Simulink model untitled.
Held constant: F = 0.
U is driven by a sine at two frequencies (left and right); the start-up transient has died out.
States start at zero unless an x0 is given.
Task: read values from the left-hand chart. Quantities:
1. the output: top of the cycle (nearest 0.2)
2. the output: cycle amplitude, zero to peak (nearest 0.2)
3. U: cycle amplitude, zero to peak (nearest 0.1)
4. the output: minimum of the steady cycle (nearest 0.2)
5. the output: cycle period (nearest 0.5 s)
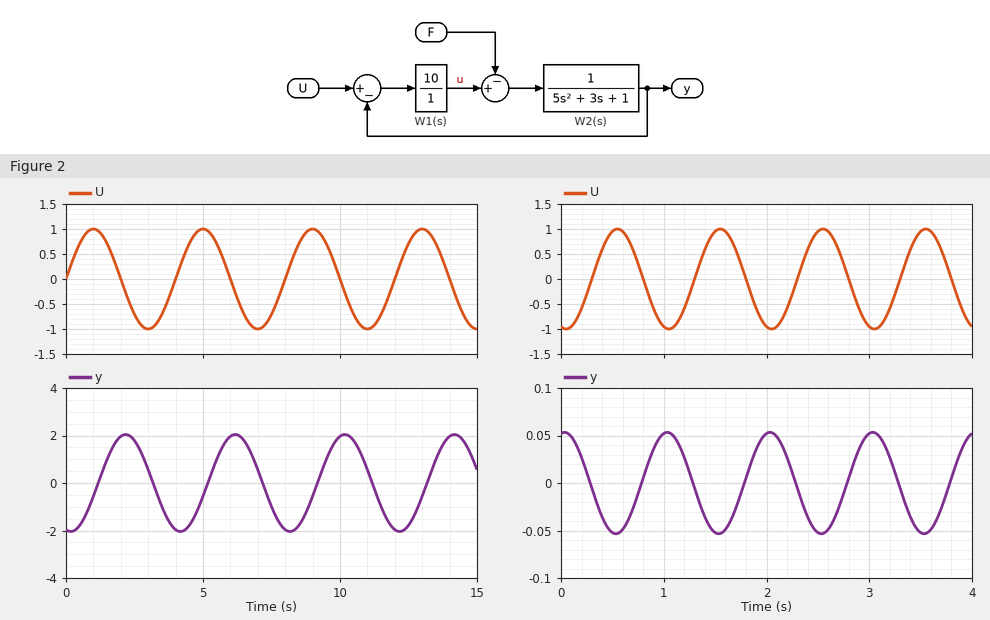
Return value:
2.0
2.0
1.0
-2.0
4.0 s
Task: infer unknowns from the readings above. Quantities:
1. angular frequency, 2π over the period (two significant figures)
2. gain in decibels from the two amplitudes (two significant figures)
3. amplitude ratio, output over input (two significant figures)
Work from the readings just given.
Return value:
1.6 rad/s
6.0 dB
2.0
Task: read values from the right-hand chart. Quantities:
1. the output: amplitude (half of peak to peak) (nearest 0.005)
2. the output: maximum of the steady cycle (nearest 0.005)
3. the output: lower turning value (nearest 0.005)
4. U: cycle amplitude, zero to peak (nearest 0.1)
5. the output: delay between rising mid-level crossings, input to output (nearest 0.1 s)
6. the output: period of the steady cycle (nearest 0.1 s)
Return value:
0.055
0.055
-0.055
1.0
0.5 s
1.0 s
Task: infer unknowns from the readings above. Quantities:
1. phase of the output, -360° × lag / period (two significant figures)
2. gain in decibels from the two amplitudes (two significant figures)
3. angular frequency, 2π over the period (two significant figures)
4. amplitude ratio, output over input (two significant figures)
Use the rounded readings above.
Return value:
-180°
-25 dB
6.3 rad/s
0.055
